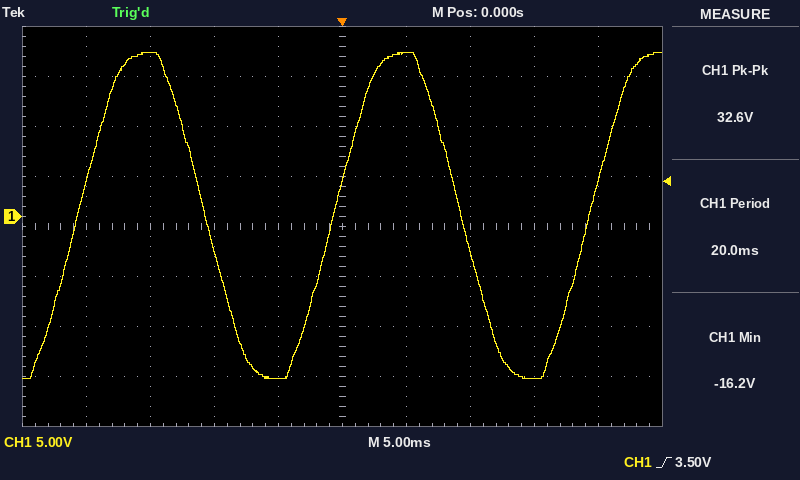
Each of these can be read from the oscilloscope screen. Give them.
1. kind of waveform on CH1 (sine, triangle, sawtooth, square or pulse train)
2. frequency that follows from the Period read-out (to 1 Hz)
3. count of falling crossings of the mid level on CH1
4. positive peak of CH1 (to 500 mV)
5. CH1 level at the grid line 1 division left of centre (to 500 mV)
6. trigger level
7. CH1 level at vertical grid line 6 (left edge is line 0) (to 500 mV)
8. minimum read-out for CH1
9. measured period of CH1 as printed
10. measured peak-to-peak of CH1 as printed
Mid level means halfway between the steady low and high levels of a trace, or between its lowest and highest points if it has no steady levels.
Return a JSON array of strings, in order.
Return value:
["sine", "50 Hz", "2", "16.5 V", "-16.0 V", "3.50 V", "16.5 V", "-16.2 V", "20.0 ms", "32.6 V"]
